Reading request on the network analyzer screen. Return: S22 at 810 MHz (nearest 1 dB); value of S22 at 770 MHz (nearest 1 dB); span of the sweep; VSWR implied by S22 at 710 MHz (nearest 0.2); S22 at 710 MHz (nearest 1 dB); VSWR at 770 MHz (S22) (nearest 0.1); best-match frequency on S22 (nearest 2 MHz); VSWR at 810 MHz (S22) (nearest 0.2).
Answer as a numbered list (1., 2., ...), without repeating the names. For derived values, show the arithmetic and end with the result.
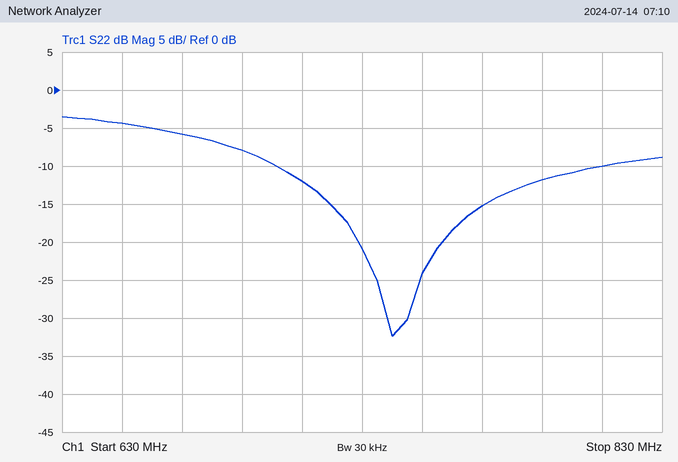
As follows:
1. -10 dB
2. -15 dB
3. 200 MHz
4. |Γ| = 10^(-12/20) = 0.2512; VSWR = (1 + 0.2512)/(1 − 0.2512) ≈ 1.67, so 1.6 to the nearest 0.2
5. -12 dB
6. |Γ| = 10^(-15/20) = 0.1778; VSWR = (1 + 0.1778)/(1 − 0.1778) ≈ 1.4
7. 740 MHz
8. |Γ| = 10^(-10/20) = 0.3162; VSWR = (1 + 0.3162)/(1 − 0.3162) ≈ 1.92, so 2.0 to the nearest 0.2
